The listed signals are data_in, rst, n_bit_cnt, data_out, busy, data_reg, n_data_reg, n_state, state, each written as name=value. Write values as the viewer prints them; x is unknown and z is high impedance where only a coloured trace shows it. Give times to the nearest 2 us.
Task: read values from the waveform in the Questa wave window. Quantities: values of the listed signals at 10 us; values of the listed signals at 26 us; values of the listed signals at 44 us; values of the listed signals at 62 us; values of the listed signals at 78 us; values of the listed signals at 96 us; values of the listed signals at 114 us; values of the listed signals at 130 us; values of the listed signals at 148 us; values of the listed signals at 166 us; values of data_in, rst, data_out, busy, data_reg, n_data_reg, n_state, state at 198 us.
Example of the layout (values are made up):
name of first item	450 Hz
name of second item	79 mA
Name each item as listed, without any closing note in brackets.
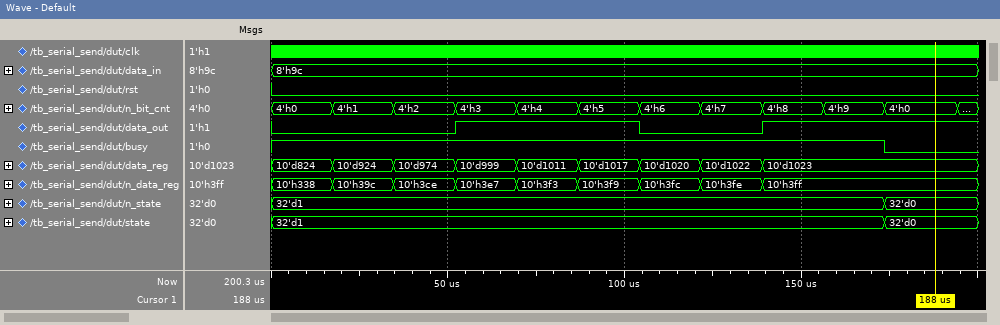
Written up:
values of the listed signals at 10 us	data_in=8'h9c, rst=0, n_bit_cnt=4'h0, data_out=0, busy=1, data_reg=10'd824, n_data_reg=10'h338, n_state=32'd1, state=32'd1
values of the listed signals at 26 us	data_in=8'h9c, rst=0, n_bit_cnt=4'h1, data_out=0, busy=1, data_reg=10'd924, n_data_reg=10'h39c, n_state=32'd1, state=32'd1
values of the listed signals at 44 us	data_in=8'h9c, rst=0, n_bit_cnt=4'h2, data_out=0, busy=1, data_reg=10'd974, n_data_reg=10'h3ce, n_state=32'd1, state=32'd1
values of the listed signals at 62 us	data_in=8'h9c, rst=0, n_bit_cnt=4'h3, data_out=1, busy=1, data_reg=10'd999, n_data_reg=10'h3e7, n_state=32'd1, state=32'd1
values of the listed signals at 78 us	data_in=8'h9c, rst=0, n_bit_cnt=4'h4, data_out=1, busy=1, data_reg=10'd1011, n_data_reg=10'h3f3, n_state=32'd1, state=32'd1
values of the listed signals at 96 us	data_in=8'h9c, rst=0, n_bit_cnt=4'h5, data_out=1, busy=1, data_reg=10'd1017, n_data_reg=10'h3f9, n_state=32'd1, state=32'd1
values of the listed signals at 114 us	data_in=8'h9c, rst=0, n_bit_cnt=4'h6, data_out=0, busy=1, data_reg=10'd1020, n_data_reg=10'h3fc, n_state=32'd1, state=32'd1
values of the listed signals at 130 us	data_in=8'h9c, rst=0, n_bit_cnt=4'h7, data_out=0, busy=1, data_reg=10'd1022, n_data_reg=10'h3fe, n_state=32'd1, state=32'd1
values of the listed signals at 148 us	data_in=8'h9c, rst=0, n_bit_cnt=4'h8, data_out=1, busy=1, data_reg=10'd1023, n_data_reg=10'h3ff, n_state=32'd1, state=32'd1
values of the listed signals at 166 us	data_in=8'h9c, rst=0, n_bit_cnt=4'h9, data_out=1, busy=1, data_reg=10'd1023, n_data_reg=10'h3ff, n_state=32'd1, state=32'd1
values of data_in, rst, data_out, busy, data_reg, n_data_reg, n_state, state at 198 us	data_in=8'h9c, rst=0, data_out=1, busy=0, data_reg=10'd1023, n_data_reg=10'h3ff, n_state=32'd0, state=32'd0
